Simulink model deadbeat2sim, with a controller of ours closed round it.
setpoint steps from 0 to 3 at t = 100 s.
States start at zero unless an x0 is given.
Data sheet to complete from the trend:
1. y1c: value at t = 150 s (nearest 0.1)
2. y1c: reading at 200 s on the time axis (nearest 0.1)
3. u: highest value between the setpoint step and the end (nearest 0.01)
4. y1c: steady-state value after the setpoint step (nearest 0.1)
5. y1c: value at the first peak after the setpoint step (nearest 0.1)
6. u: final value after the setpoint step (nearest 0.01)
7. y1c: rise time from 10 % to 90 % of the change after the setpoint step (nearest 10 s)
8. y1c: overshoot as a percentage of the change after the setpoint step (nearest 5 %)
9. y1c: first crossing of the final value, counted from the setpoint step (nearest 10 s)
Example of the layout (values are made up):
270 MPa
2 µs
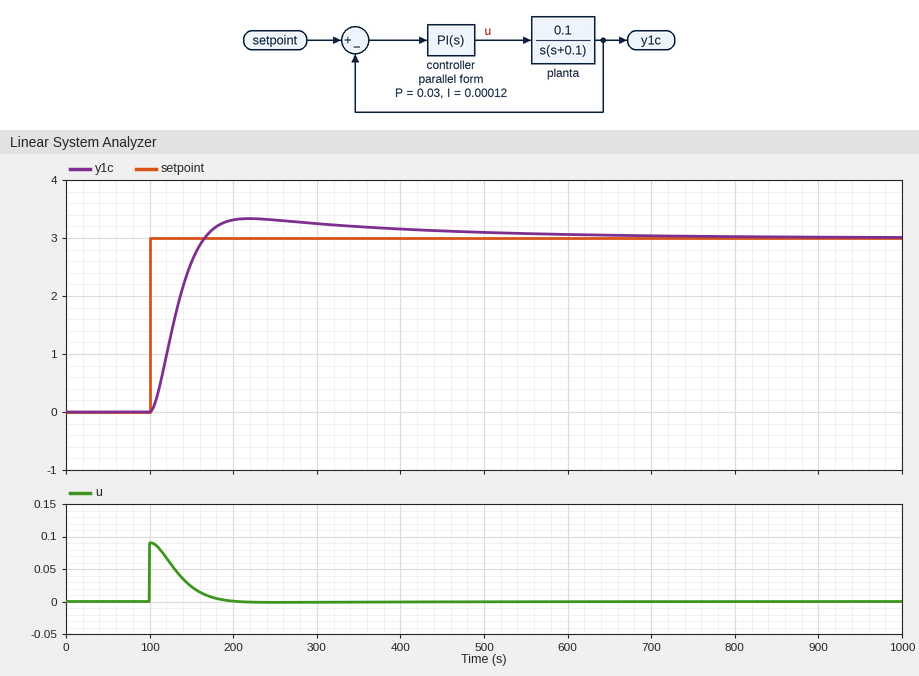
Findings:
2.6
3.3
0.09
3.0
3.3
0.00
40 s
10 %
70 s
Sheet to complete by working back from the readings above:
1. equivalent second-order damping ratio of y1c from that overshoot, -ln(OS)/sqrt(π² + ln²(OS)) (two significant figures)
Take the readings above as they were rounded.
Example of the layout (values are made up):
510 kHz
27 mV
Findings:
0.59
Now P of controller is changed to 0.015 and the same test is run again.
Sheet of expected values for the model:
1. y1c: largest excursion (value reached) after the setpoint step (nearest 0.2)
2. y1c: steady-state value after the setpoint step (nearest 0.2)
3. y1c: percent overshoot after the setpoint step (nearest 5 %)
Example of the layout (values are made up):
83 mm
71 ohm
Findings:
3.8
3.0
25 %
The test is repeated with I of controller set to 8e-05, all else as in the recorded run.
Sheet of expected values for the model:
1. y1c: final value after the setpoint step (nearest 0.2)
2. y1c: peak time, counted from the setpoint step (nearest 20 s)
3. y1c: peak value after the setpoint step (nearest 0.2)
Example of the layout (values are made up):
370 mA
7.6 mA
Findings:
3.0
120 s
3.2
